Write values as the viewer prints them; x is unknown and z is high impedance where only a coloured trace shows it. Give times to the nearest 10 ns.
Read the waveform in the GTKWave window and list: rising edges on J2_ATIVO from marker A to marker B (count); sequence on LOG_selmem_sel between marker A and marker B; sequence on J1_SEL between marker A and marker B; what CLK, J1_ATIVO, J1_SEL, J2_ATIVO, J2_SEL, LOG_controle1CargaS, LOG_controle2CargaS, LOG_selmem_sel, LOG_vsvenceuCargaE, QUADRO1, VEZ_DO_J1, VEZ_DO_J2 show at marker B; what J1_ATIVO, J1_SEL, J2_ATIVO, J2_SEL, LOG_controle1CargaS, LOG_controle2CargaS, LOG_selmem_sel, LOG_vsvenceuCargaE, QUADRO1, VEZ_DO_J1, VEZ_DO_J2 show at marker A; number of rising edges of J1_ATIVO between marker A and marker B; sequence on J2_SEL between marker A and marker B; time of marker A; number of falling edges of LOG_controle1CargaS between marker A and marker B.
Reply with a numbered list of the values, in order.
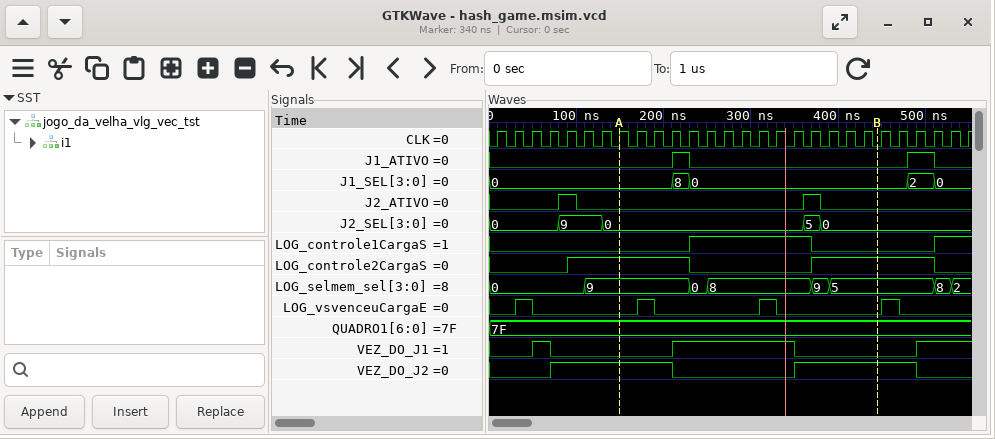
1. 1
2. 9, 0, 8, 9, 5
3. 0, 8, 0
4. CLK=0, J1_ATIVO=0, J1_SEL=0, J2_ATIVO=0, J2_SEL=0, LOG_controle1CargaS=0, LOG_controle2CargaS=1, LOG_selmem_sel=5, LOG_vsvenceuCargaE=0, QUADRO1=7F, VEZ_DO_J1=0, VEZ_DO_J2=1
5. J1_ATIVO=0, J1_SEL=0, J2_ATIVO=0, J2_SEL=0, LOG_controle1CargaS=0, LOG_controle2CargaS=1, LOG_selmem_sel=9, LOG_vsvenceuCargaE=0, QUADRO1=7F, VEZ_DO_J1=0, VEZ_DO_J2=1
6. 1
7. 0, 5, 0
8. 150 ns
9. 1
